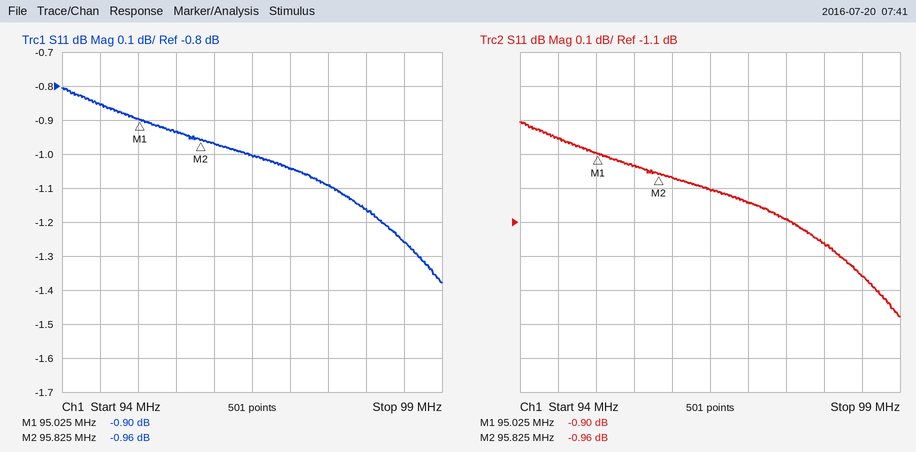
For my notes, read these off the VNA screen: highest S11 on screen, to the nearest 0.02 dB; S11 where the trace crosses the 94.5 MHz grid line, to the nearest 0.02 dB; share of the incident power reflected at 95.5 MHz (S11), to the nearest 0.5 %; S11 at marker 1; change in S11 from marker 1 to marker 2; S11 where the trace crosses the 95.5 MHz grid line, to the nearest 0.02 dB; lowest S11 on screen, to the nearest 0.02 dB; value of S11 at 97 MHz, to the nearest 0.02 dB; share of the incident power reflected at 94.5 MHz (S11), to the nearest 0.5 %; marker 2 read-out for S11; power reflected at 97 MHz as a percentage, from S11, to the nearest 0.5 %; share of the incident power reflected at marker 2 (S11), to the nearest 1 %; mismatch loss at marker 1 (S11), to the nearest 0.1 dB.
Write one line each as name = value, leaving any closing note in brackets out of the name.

highest S11 on screen, to the nearest 0.02 dB = -0.80 dB
S11 where the trace crosses the 94.5 MHz grid line, to the nearest 0.02 dB = -0.86 dB
share of the incident power reflected at 95.5 MHz (S11), to the nearest 0.5 % = 80.5 %
S11 at marker 1 = -0.90 dB
change in S11 from marker 1 to marker 2 = -0.06 dB
S11 where the trace crosses the 95.5 MHz grid line, to the nearest 0.02 dB = -0.94 dB
lowest S11 on screen, to the nearest 0.02 dB = -1.38 dB
value of S11 at 97 MHz, to the nearest 0.02 dB = -1.04 dB
share of the incident power reflected at 94.5 MHz (S11), to the nearest 0.5 % = 82.0 %
marker 2 read-out for S11 = -0.96 dB
power reflected at 97 MHz as a percentage, from S11, to the nearest 0.5 % = 78.5 %
share of the incident power reflected at marker 2 (S11), to the nearest 1 % = 80 %
mismatch loss at marker 1 (S11), to the nearest 0.1 dB = 7.3 dB
